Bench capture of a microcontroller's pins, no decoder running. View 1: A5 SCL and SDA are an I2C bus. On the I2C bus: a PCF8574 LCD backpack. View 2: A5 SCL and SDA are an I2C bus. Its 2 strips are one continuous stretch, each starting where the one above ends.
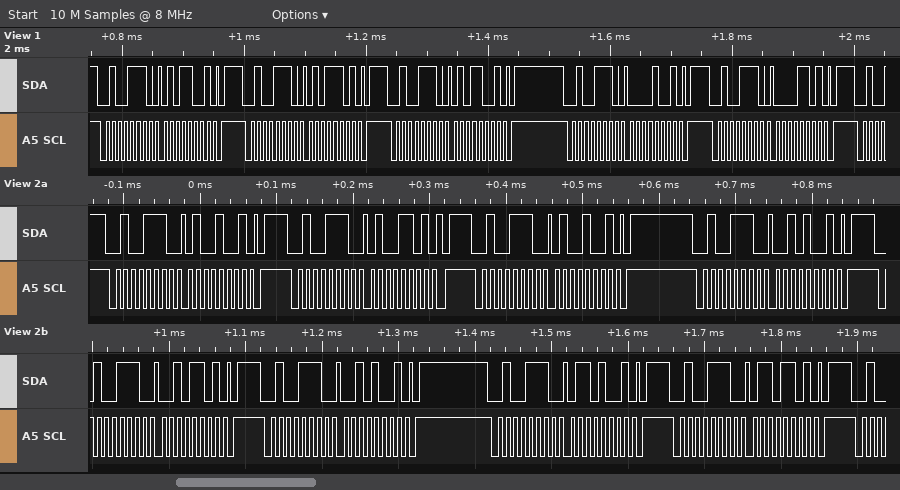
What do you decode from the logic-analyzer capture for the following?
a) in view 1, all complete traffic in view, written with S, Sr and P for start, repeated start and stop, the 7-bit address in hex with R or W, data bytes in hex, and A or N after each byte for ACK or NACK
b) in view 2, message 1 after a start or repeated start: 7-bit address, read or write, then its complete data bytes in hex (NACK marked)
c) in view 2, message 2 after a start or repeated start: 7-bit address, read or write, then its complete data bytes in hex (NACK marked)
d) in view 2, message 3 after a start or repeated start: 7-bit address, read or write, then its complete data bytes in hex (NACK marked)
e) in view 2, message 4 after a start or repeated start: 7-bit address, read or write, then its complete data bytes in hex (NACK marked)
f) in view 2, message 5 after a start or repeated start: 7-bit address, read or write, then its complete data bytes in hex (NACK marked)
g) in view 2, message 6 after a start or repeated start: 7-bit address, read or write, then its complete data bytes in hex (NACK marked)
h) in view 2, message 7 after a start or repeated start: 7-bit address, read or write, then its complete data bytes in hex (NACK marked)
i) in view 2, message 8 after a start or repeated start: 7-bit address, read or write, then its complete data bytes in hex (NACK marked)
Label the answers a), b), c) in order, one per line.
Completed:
a) S 27W A 59 A P S 27W A 5D A P S 27W A 59 A P S 27W A 09 A P S 27W A 0D A P
b) 0x27 write: 49
c) 0x27 write: 4D
d) 0x27 write: 49
e) 0x27 write: 29
f) 0x27 write: 2D
g) 0x27 write: 29
h) 0x27 write: 69
i) 0x27 write: 6D
